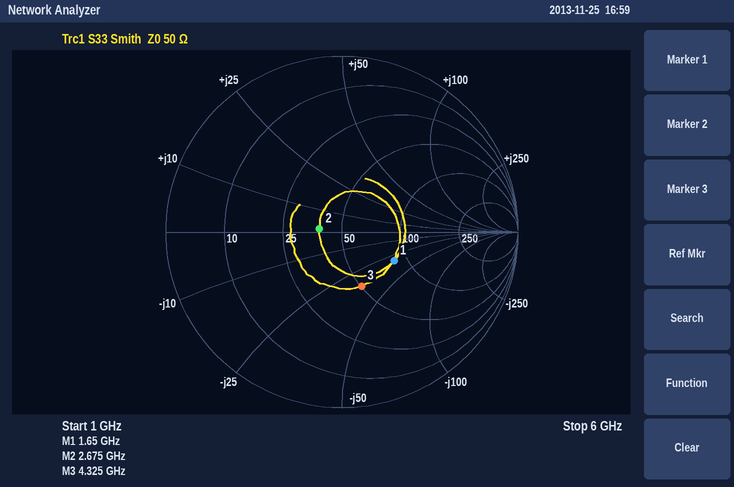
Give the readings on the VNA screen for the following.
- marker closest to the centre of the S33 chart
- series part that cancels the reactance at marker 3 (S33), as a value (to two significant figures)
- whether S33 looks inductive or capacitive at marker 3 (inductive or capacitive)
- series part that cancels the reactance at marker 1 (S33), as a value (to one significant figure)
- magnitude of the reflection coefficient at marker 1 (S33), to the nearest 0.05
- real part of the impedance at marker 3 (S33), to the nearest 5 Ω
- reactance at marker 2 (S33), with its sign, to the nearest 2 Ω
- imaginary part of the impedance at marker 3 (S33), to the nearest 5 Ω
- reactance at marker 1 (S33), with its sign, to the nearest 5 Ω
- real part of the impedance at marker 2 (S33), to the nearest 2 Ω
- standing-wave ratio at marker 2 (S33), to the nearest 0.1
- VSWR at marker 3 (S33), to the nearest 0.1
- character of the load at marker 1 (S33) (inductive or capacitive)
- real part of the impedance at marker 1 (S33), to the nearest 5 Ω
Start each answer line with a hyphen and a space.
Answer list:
- marker 2
- 1.3 nH
- capacitive
- 3 nH
- 0.35
- 50 Ω
- +2 Ω
- -35 Ω
- -30 Ω
- 38 Ω
- 1.3
- 2.0
- capacitive
- 85 Ω
